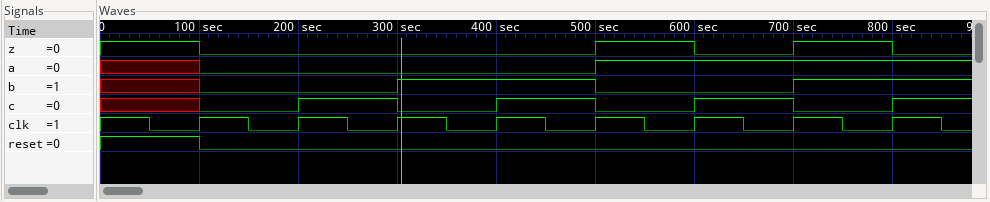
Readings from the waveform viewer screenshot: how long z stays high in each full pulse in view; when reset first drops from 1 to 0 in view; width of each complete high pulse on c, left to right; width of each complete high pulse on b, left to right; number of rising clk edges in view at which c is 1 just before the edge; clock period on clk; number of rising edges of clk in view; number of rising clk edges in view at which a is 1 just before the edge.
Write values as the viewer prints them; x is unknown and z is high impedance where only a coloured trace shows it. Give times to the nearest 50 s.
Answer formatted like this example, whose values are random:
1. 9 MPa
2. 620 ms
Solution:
1. 100 s, 100 s
2. 100 s
3. 100 s, 100 s, 100 s
4. 200 s
5. 3
6. 100 s
7. 8
8. 3
